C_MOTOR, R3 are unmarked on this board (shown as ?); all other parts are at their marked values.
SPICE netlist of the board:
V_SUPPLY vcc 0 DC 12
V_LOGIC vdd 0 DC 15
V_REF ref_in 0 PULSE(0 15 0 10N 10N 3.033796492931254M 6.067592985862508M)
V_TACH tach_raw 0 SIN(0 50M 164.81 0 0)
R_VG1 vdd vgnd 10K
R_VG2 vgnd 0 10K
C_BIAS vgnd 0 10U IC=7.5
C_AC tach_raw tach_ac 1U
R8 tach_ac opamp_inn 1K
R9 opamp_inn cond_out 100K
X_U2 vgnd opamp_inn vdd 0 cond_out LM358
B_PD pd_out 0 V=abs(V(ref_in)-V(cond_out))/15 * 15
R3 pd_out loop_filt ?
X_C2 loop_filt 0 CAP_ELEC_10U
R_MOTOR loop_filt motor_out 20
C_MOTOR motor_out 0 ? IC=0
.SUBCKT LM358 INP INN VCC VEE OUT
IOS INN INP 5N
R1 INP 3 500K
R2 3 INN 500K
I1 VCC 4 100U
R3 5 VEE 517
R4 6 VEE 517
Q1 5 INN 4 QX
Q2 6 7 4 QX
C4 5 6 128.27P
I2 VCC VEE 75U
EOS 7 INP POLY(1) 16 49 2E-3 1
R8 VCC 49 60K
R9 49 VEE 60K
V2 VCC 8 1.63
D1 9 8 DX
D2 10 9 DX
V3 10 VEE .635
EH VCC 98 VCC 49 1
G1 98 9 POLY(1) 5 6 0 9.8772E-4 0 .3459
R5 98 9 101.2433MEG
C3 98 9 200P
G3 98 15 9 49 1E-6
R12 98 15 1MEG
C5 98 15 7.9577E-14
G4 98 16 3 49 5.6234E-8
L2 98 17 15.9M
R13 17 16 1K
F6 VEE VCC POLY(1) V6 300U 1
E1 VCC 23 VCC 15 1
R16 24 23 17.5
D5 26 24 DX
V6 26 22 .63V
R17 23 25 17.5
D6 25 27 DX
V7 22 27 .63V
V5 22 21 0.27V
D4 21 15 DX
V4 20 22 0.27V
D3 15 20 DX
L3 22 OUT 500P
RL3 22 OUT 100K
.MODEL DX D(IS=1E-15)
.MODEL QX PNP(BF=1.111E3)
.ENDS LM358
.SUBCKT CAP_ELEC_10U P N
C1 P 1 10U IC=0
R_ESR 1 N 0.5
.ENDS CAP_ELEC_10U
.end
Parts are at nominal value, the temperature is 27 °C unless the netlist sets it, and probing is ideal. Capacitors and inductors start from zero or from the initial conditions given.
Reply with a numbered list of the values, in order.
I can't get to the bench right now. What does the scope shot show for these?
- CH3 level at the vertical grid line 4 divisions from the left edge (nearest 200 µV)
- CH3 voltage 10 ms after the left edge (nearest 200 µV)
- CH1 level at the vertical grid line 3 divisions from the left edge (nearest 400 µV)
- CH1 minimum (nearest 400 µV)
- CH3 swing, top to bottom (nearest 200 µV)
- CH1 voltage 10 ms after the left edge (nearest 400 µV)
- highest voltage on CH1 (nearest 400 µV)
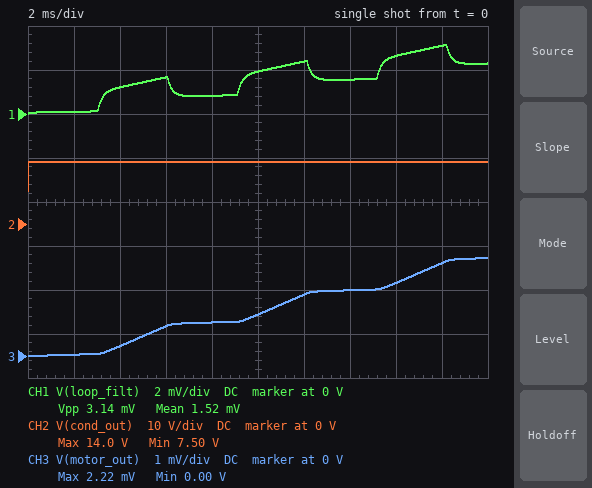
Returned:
1. 800 µV
2. 1.0 mV
3. 1.6 mV
4. 0 V
5. 2.2 mV
6. 2.0 mV
7. 3.2 mV
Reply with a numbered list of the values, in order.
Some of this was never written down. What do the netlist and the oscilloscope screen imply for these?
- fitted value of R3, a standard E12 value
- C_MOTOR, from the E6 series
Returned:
1. 270 kΩ
2. 220 µF
